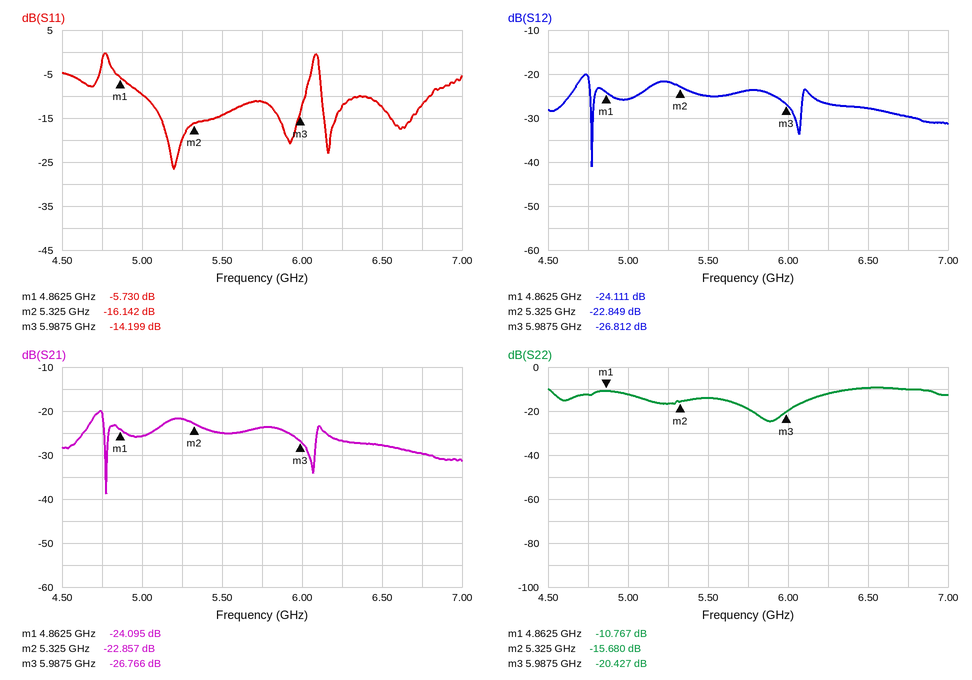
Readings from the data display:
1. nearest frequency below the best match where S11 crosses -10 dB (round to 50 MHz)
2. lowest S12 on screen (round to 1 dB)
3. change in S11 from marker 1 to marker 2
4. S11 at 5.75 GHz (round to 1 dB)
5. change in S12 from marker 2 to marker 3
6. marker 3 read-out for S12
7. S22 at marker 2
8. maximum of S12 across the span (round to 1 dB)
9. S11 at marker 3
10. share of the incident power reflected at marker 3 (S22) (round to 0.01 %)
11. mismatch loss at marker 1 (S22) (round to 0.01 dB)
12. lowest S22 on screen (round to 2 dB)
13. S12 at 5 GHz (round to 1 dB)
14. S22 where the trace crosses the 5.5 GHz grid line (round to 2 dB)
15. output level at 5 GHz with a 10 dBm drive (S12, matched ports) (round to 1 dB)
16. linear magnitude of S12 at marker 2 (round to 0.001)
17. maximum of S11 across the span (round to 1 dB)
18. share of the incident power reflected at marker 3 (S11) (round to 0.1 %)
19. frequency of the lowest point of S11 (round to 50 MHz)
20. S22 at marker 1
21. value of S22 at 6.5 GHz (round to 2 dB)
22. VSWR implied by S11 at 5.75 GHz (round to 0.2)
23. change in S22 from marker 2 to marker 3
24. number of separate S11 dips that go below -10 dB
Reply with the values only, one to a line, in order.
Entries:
5.00 GHz
-41 dB
-10.412 dB
-11 dB
-3.963 dB
-26.812 dB
-15.680 dB
-20 dB
-14.199 dB
0.91 %
0.38 dB
-24 dB
-26 dB
-14 dB
-16 dBm
0.072
0 dB
3.8 %
5.20 GHz
-10.767 dB
-10 dB
1.8
-4.747 dB
4
